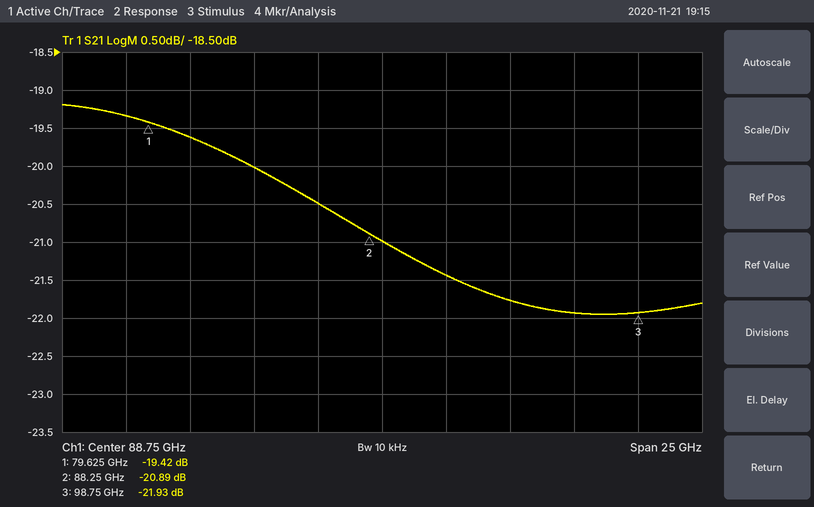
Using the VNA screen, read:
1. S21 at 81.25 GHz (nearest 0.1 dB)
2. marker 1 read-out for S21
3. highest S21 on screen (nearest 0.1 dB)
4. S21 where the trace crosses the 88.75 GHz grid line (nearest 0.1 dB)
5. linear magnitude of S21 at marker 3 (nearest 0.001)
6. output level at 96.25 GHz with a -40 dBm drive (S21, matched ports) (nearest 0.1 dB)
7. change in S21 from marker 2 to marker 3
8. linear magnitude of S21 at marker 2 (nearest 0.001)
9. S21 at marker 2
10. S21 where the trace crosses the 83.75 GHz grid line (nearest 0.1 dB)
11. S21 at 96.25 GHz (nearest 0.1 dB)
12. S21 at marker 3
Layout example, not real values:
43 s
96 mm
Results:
-19.6 dB
-19.42 dB
-19.2 dB
-21.0 dB
0.080
-61.9 dBm
-1.04 dB
0.090
-20.89 dB
-20.0 dB
-21.9 dB
-21.93 dB
